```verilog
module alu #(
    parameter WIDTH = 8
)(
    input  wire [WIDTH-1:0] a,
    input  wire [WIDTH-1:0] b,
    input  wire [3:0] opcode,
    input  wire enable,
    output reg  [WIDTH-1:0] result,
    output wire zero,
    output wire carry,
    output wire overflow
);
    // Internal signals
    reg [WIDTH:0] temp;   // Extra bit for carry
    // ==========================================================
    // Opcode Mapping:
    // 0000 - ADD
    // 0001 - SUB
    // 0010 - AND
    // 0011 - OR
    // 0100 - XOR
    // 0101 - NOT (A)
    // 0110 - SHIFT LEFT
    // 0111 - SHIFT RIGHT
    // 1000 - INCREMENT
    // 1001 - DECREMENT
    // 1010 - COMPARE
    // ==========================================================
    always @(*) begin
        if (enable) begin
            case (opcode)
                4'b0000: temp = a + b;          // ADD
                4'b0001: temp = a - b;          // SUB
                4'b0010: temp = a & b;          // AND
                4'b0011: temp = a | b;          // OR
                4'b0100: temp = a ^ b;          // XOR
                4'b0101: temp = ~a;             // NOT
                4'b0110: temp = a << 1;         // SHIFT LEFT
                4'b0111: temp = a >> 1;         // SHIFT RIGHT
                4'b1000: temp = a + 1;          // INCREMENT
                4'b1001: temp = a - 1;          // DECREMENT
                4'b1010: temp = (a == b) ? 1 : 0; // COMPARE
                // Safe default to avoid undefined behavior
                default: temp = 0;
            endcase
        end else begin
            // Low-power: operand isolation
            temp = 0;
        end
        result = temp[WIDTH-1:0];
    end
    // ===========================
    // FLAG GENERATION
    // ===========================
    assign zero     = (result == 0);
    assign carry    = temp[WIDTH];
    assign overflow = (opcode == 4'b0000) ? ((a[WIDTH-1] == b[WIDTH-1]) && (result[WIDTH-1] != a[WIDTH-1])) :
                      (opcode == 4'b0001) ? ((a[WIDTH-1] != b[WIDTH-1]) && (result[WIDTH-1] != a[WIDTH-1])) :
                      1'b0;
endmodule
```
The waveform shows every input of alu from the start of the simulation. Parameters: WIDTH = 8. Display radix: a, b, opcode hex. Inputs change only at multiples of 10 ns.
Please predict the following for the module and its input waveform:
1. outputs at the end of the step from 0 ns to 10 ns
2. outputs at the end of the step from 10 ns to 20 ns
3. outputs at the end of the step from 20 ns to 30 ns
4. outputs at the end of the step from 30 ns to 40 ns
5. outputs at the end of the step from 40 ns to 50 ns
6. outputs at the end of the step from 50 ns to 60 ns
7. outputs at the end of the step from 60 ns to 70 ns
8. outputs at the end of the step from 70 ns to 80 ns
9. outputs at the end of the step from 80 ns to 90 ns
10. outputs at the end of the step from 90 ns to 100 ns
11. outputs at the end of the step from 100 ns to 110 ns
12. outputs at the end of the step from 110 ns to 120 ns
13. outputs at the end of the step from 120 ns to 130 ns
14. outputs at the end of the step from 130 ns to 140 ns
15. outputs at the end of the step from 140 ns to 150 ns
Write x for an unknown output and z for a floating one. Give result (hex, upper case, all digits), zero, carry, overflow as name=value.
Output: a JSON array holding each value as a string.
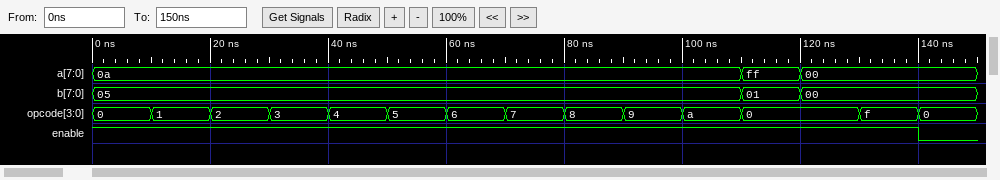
["result=0F, zero=0, carry=0, overflow=0", "result=05, zero=0, carry=0, overflow=0", "result=00, zero=1, carry=0, overflow=0", "result=0F, zero=0, carry=0, overflow=0", "result=0F, zero=0, carry=0, overflow=0", "result=F5, zero=0, carry=1, overflow=0", "result=14, zero=0, carry=0, overflow=0", "result=05, zero=0, carry=0, overflow=0", "result=0B, zero=0, carry=0, overflow=0", "result=09, zero=0, carry=0, overflow=0", "result=00, zero=1, carry=0, overflow=0", "result=00, zero=1, carry=1, overflow=0", "result=00, zero=1, carry=0, overflow=0", "result=00, zero=1, carry=0, overflow=0", "result=00, zero=1, carry=0, overflow=0"]
